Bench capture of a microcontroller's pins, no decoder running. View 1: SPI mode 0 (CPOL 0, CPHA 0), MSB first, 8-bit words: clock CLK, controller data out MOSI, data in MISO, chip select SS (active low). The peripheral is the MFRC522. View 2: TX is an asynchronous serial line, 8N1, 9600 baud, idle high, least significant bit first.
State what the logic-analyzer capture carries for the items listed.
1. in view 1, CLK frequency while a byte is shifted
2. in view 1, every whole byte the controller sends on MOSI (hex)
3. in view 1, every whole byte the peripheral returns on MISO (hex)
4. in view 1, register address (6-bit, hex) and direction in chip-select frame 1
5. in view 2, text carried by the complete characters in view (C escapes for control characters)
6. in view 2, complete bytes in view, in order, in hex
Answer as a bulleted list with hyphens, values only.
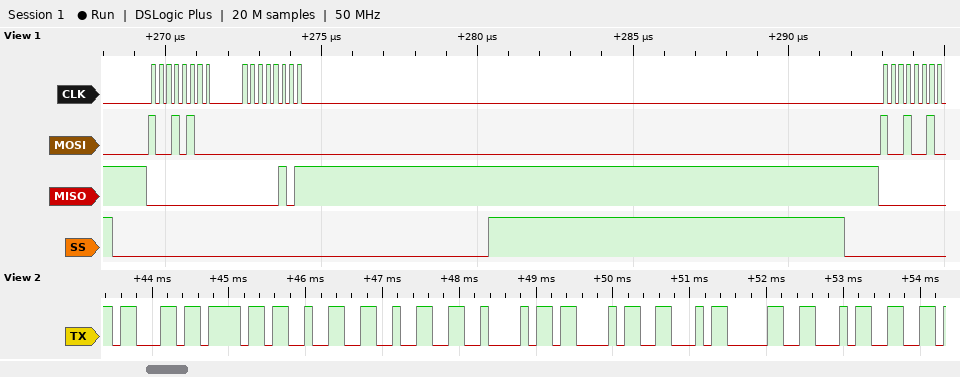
- 4 MHz
- 0x94 0x00 0x92
- 0x00 0x05 0x00
- 0x0A read
- "co22BCF04"
- 0x63 0x6F 0x32 0x32 0x42 0x43 0x46 0x30 0x34
